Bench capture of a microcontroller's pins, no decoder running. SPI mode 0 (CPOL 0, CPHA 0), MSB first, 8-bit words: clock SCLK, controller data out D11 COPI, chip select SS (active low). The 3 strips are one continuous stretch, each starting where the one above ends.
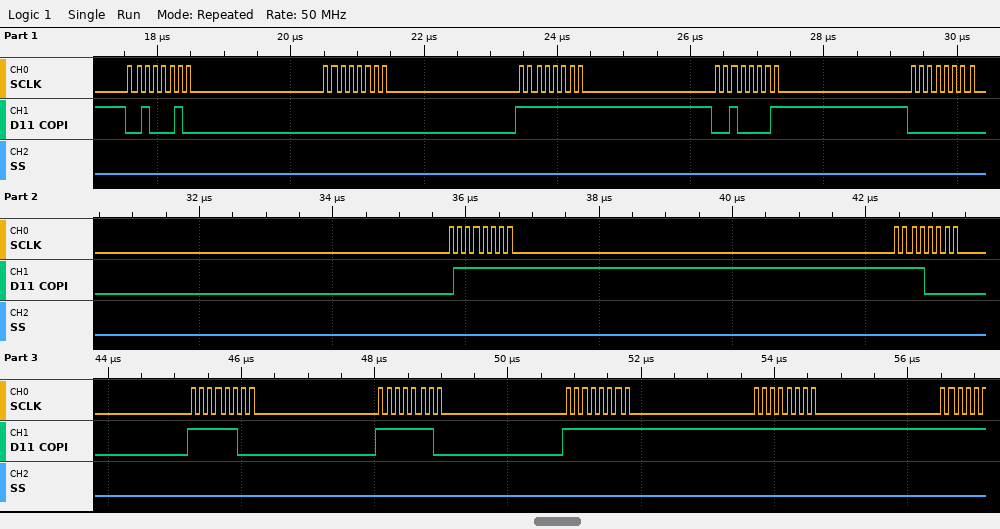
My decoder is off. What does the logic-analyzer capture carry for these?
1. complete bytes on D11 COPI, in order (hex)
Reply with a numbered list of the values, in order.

1. 22 00 FF 21 00 7F F0 FC FE FF FF
